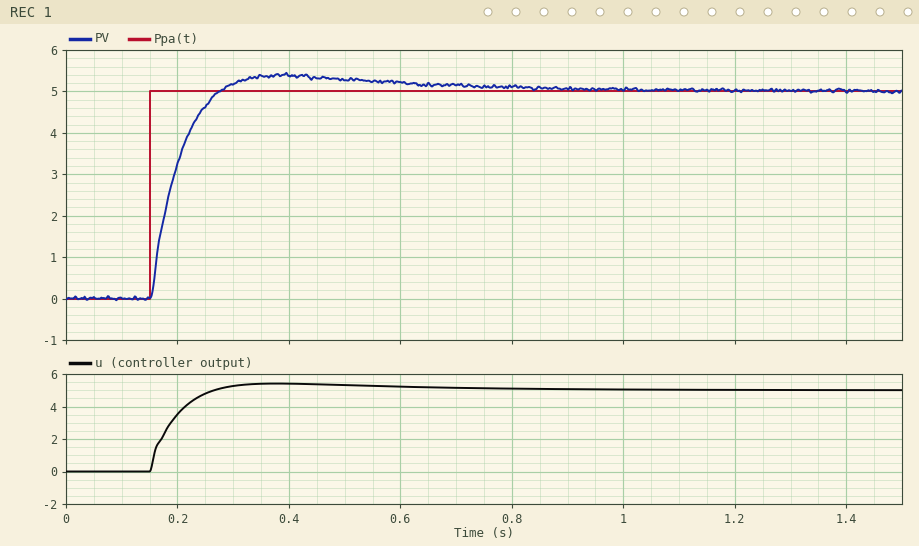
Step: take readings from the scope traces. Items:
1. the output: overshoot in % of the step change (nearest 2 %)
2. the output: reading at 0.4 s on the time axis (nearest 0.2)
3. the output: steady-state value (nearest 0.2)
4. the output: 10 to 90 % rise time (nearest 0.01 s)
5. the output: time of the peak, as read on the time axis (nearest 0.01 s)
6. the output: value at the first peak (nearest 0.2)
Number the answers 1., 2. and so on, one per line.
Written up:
1. 8 %
2. 5.4
3. 5.0
4. 0.08 s
5. 0.39 s
6. 5.4
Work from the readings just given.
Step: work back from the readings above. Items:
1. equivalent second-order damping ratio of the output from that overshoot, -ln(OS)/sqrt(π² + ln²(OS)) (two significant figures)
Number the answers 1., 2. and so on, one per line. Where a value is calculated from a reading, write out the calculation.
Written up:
1. ln(0.08) = -2.526; 2.526 / sqrt(9.870 + 6.379) = 0.63
